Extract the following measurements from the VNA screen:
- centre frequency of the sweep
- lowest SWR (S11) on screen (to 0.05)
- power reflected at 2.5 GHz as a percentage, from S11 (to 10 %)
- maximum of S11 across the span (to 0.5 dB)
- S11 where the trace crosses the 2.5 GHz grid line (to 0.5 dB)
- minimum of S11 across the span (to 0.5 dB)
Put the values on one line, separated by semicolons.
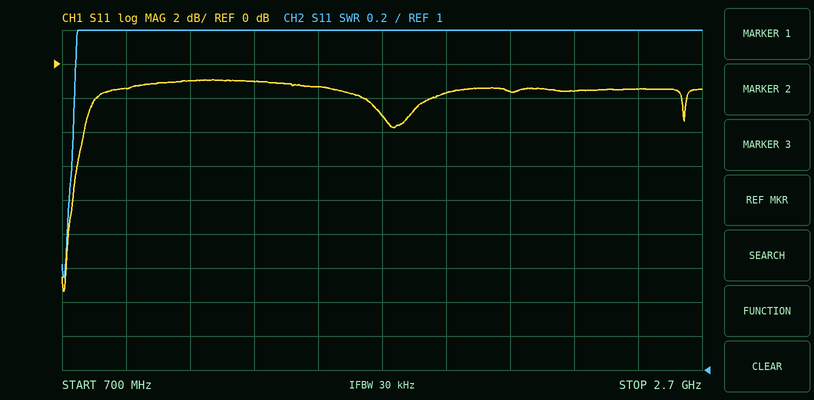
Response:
1.7 GHz; 1.55; 70 %; -1.0 dB; -1.5 dB; -13.5 dB
